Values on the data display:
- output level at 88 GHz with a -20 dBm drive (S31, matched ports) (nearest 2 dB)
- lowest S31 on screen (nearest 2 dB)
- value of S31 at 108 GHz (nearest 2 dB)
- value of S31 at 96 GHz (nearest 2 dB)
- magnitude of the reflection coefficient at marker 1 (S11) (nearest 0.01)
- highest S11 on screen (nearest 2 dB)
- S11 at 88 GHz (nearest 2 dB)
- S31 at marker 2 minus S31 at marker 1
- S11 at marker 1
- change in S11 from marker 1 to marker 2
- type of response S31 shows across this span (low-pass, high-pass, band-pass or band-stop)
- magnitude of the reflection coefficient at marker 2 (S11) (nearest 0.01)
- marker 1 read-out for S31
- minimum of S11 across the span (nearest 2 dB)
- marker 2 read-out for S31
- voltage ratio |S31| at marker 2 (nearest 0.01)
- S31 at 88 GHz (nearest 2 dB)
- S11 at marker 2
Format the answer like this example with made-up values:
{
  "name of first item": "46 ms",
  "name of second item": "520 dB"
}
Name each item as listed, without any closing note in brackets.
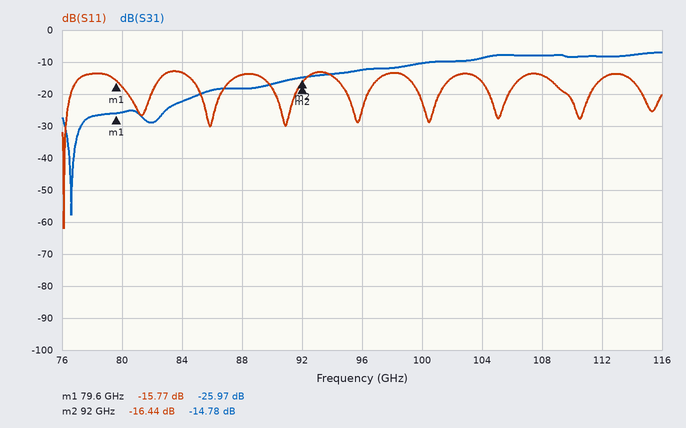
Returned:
{
  "output level at 88 GHz with a -20 dBm drive (S31, matched ports)": "-38 dBm",
  "lowest S31 on screen": "-58 dB",
  "value of S31 at 108 GHz": "-8 dB",
  "value of S31 at 96 GHz": "-12 dB",
  "magnitude of the reflection coefficient at marker 1 (S11)": "0.16",
  "highest S11 on screen": "-12 dB",
  "S11 at 88 GHz": "-14 dB",
  "S31 at marker 2 minus S31 at marker 1": "11.19 dB",
  "S11 at marker 1": "-15.77 dB",
  "change in S11 from marker 1 to marker 2": "-0.67 dB",
  "type of response S31 shows across this span": "high-pass",
  "magnitude of the reflection coefficient at marker 2 (S11)": "0.15",
  "marker 1 read-out for S31": "-25.97 dB",
  "minimum of S11 across the span": "-62 dB",
  "marker 2 read-out for S31": "-14.78 dB",
  "voltage ratio |S31| at marker 2": "0.18",
  "S31 at 88 GHz": "-18 dB",
  "S11 at marker 2": "-16.44 dB"
}
